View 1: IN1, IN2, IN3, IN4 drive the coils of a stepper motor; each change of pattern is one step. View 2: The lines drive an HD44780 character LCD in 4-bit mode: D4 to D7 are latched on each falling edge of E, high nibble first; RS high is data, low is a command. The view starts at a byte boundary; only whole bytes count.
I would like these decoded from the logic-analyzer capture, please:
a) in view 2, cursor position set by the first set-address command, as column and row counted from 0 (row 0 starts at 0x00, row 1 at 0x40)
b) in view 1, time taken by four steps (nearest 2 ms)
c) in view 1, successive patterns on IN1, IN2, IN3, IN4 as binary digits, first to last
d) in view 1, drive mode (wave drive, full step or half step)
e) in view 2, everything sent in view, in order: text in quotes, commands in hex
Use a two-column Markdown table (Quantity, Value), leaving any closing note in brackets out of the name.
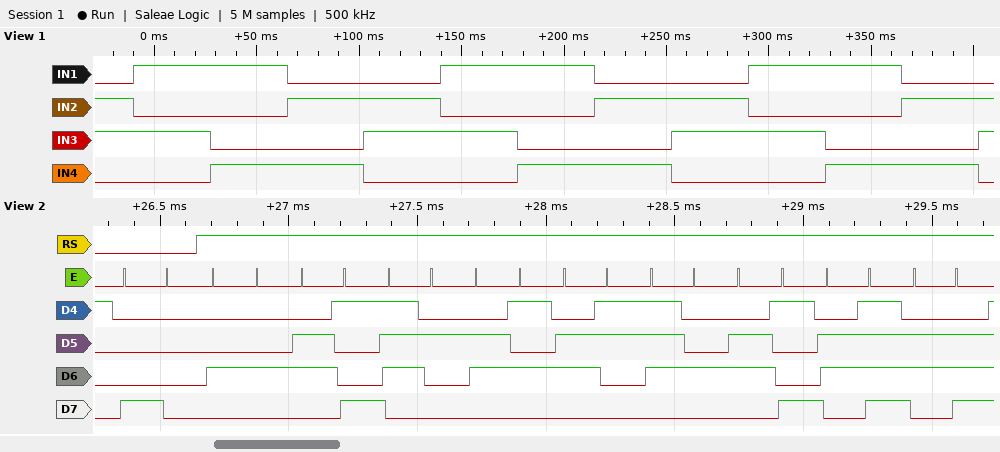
| Quantity | Value |
|---|---|
| in view 2, cursor position set by the first set-address command, as column and row counted from 0 | column 0, row 0 |
| in view 1, time taken by four steps | 150 ms |
| in view 1, successive patterns on IN1, IN2, IN3, IN4 as binary digits, first to last | 0110 1010 1001 0101 0110 1010 1001 0101 0110 1010 1001 0101 0110 |
| in view 1, drive mode | full step |
| in view 2, everything sent in view, in order: text in quotes, commands in hex | 0x80 "Direction" |
